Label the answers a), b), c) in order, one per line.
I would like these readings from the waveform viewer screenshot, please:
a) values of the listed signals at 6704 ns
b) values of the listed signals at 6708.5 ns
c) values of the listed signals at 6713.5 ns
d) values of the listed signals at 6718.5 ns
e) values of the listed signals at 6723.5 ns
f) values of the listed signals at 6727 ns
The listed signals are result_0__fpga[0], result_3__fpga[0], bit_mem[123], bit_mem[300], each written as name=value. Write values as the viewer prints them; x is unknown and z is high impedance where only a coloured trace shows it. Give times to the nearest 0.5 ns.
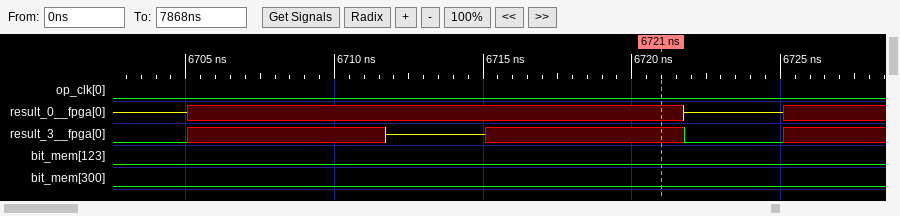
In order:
a) result_0__fpga[0]=z, result_3__fpga[0]=0, bit_mem[123]=0, bit_mem[300]=0
b) result_0__fpga[0]=x, result_3__fpga[0]=x, bit_mem[123]=0, bit_mem[300]=0
c) result_0__fpga[0]=x, result_3__fpga[0]=z, bit_mem[123]=0, bit_mem[300]=0
d) result_0__fpga[0]=x, result_3__fpga[0]=x, bit_mem[123]=0, bit_mem[300]=0
e) result_0__fpga[0]=z, result_3__fpga[0]=0, bit_mem[123]=0, bit_mem[300]=0
f) result_0__fpga[0]=x, result_3__fpga[0]=x, bit_mem[123]=0, bit_mem[300]=0
